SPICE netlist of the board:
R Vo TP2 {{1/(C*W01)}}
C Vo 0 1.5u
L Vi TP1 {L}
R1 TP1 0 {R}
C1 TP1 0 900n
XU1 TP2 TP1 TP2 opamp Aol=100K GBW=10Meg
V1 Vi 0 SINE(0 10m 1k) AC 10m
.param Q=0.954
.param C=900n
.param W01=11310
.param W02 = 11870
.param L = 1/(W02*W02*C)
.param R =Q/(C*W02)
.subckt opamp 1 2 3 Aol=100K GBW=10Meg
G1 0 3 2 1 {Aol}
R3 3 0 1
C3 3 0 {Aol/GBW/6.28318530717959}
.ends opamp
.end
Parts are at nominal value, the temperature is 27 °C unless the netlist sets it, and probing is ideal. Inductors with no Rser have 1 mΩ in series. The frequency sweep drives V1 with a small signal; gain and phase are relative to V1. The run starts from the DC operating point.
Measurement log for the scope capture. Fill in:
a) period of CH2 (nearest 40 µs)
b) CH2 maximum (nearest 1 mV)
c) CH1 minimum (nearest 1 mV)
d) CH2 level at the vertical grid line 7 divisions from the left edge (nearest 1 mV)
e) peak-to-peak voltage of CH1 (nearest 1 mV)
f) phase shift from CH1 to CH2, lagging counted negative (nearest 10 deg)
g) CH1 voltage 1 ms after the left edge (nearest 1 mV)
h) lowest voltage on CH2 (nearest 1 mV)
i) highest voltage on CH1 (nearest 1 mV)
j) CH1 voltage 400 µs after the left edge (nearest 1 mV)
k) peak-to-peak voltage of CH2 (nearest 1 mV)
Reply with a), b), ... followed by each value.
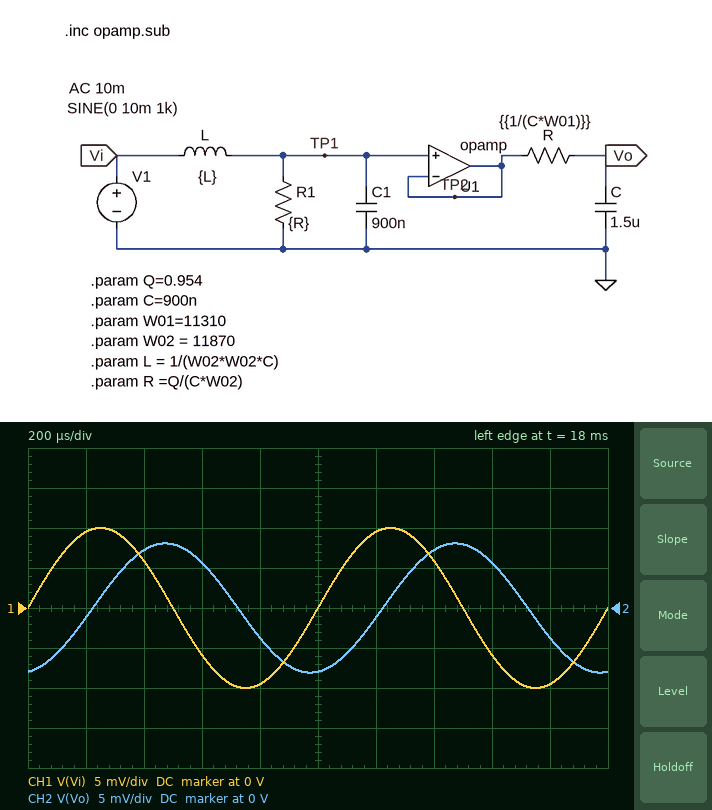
a) 1.00 ms
b) 8 mV
c) -10 mV
d) 7 mV
e) 20 mV
f) -80 deg
g) 0 V
h) -8 mV
i) 10 mV
j) 6 mV
k) 16 mV
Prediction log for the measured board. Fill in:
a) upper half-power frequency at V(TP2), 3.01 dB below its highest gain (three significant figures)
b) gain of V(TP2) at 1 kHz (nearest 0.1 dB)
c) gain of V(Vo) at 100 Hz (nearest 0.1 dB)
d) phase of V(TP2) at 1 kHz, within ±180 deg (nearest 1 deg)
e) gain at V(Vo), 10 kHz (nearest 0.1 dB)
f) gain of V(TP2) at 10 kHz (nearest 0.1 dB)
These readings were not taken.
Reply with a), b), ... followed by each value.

a) 2.19 kHz
b) 0.8 dB
c) 0 dB
d) -38 deg
e) -48.2 dB
f) -28.8 dB
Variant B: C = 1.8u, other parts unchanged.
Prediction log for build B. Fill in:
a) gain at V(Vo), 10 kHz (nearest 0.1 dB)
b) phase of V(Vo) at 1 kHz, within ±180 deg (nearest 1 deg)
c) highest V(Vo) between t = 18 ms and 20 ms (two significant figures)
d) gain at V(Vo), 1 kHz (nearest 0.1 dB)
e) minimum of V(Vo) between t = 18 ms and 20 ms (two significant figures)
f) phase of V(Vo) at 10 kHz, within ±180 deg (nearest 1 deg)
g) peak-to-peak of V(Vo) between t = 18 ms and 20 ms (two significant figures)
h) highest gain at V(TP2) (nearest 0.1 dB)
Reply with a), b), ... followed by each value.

a) -49.8 dB
b) -86 deg
c) 7.4 mV
d) -2.7 dB
e) -7.4 mV
f) 107 deg
g) 15 mV
h) 1.0 dB
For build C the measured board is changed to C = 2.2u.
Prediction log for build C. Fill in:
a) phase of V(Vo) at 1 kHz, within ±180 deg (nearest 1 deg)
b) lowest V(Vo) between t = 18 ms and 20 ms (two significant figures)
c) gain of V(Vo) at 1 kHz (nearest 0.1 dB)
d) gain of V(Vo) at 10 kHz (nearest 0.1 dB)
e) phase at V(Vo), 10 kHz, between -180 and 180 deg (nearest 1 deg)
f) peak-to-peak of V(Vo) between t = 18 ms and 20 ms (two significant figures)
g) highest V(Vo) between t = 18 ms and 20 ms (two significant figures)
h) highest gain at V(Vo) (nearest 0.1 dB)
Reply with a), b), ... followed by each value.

a) -91 deg
b) -6.5 mV
c) -3.7 dB
d) -51.5 dB
e) 106 deg
f) 13 mV
g) 6.5 mV
h) 0 dB
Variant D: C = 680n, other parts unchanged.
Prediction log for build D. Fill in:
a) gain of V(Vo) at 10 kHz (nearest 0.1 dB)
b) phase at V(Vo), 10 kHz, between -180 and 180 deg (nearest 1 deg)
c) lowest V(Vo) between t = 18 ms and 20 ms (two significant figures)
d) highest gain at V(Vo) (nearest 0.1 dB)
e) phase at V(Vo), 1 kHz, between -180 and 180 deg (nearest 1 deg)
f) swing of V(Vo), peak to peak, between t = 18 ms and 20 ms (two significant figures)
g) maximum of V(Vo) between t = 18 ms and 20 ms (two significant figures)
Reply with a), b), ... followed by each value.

a) -41.5 dB
b) 115 deg
c) -10 mV
d) 0.1 dB
e) -60 deg
f) 20 mV
g) 10 mV
